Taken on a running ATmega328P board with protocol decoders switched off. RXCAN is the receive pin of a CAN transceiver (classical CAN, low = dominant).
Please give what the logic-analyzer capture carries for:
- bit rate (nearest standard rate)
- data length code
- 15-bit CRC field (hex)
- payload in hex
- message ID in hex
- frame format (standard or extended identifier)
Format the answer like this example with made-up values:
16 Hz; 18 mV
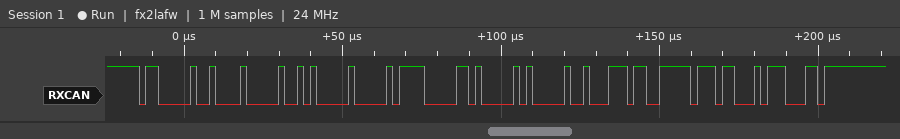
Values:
500 kbit/s; 8; 0x3171; 0A 00 3C 14 08 08 EC FF; 0x602; standard
